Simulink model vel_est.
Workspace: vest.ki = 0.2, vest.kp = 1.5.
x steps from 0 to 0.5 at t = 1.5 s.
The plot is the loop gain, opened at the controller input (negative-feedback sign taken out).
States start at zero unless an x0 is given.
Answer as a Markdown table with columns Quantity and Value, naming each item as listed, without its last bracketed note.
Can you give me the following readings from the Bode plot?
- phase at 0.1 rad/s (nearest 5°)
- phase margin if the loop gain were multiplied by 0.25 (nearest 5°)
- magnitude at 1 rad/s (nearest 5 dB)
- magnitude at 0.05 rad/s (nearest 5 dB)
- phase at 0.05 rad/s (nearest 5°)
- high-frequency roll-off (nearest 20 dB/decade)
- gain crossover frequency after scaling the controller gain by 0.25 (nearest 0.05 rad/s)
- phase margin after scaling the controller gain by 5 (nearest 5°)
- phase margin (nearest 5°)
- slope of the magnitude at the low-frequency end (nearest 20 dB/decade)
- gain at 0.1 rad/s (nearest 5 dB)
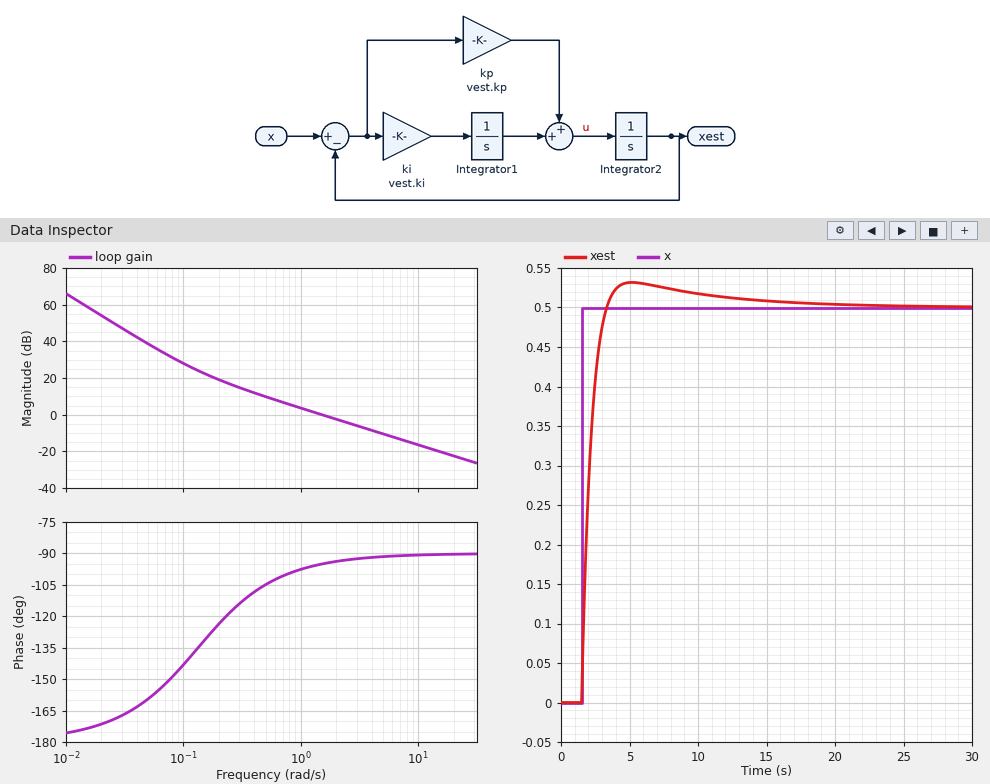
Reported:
| Quantity | Value |
|---|---|
| phase at 0.1 rad/s | -145° |
| phase margin if the loop gain were multiplied by 0.25 | 70° |
| magnitude at 1 rad/s | 5 dB |
| magnitude at 0.05 rad/s | 40 dB |
| phase at 0.05 rad/s | -160° |
| high-frequency roll-off | -20 dB/decade |
| gain crossover frequency after scaling the controller gain by 0.25 | 0.40 rad/s |
| phase margin after scaling the controller gain by 5 | 90° |
| phase margin | 85° |
| slope of the magnitude at the low-frequency end | -40 dB/decade |
| gain at 0.1 rad/s | 30 dB |
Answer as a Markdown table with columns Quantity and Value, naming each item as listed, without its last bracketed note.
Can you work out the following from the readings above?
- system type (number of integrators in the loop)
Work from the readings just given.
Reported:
| Quantity | Value |
|---|---|
| system type | 2 |
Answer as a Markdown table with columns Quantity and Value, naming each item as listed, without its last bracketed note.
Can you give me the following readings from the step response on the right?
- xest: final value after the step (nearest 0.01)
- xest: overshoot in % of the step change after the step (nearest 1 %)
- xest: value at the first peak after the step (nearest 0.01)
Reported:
| Quantity | Value |
|---|---|
| xest: final value after the step | 0.50 |
| xest: overshoot in % of the step change after the step | 6 % |
| xest: value at the first peak after the step | 0.53 |
